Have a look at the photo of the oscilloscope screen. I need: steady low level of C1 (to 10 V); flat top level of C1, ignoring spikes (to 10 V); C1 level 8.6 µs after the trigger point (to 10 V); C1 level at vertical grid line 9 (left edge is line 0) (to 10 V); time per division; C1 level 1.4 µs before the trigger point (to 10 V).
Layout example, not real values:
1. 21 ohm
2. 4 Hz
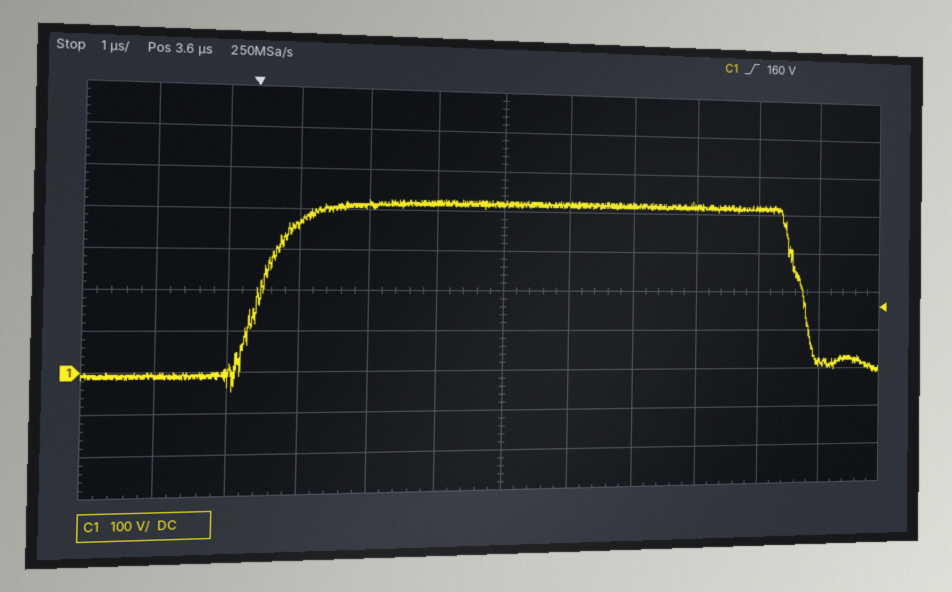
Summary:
1. -10 V
2. 420 V
3. 20 V
4. 420 V
5. 1 µs
6. -10 V
